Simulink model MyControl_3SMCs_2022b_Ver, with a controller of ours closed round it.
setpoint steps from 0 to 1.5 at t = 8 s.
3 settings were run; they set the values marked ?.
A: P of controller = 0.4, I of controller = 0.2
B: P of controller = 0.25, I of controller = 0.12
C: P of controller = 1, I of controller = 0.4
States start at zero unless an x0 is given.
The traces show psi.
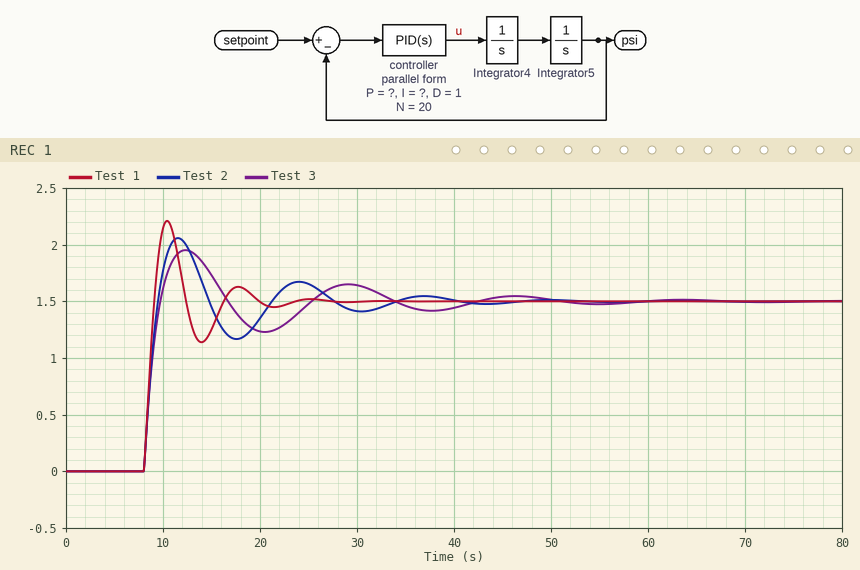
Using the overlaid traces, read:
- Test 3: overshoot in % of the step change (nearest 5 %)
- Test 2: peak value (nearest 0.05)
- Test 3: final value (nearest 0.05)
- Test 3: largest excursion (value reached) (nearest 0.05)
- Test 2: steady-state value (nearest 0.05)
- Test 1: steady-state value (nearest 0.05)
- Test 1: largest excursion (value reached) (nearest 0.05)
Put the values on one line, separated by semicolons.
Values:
30 %; 2.05; 1.50; 1.95; 1.50; 1.50; 2.20
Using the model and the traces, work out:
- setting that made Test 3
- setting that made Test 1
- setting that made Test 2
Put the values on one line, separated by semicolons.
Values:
B; C; A
